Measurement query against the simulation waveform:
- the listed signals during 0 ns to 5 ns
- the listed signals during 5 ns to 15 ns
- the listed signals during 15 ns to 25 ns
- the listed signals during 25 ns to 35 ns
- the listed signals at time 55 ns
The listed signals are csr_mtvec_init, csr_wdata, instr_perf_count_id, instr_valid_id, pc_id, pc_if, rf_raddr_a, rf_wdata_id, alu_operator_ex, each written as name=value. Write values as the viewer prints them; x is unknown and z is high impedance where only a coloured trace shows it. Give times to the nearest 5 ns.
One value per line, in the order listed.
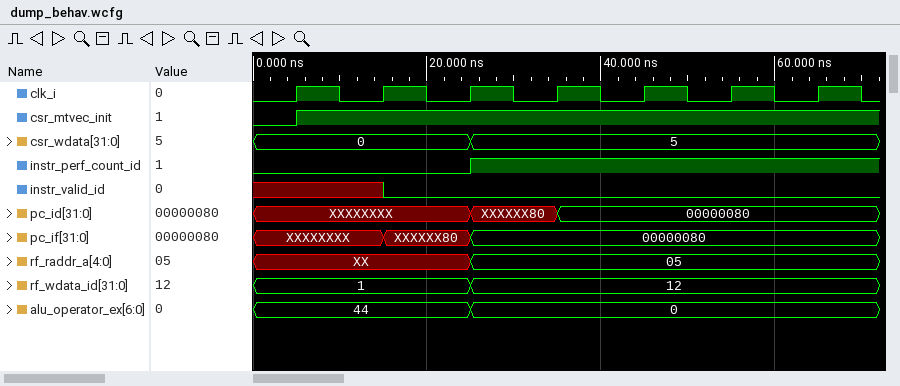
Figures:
csr_mtvec_init=0, csr_wdata=0, instr_perf_count_id=0, instr_valid_id=x, pc_id=XXXXXXXX, pc_if=XXXXXXXX, rf_raddr_a=XX, rf_wdata_id=1, alu_operator_ex=44
csr_mtvec_init=1, csr_wdata=0, instr_perf_count_id=0, instr_valid_id=x, pc_id=XXXXXXXX, pc_if=XXXXXXXX, rf_raddr_a=XX, rf_wdata_id=1, alu_operator_ex=44
csr_mtvec_init=1, csr_wdata=0, instr_perf_count_id=0, instr_valid_id=0, pc_id=XXXXXXXX, pc_if=XXXXXX80, rf_raddr_a=XX, rf_wdata_id=1, alu_operator_ex=44
csr_mtvec_init=1, csr_wdata=5, instr_perf_count_id=1, instr_valid_id=0, pc_id=XXXXXX80, pc_if=00000080, rf_raddr_a=05, rf_wdata_id=12, alu_operator_ex=0
csr_mtvec_init=1, csr_wdata=5, instr_perf_count_id=1, instr_valid_id=0, pc_id=00000080, pc_if=00000080, rf_raddr_a=05, rf_wdata_id=12, alu_operator_ex=0
